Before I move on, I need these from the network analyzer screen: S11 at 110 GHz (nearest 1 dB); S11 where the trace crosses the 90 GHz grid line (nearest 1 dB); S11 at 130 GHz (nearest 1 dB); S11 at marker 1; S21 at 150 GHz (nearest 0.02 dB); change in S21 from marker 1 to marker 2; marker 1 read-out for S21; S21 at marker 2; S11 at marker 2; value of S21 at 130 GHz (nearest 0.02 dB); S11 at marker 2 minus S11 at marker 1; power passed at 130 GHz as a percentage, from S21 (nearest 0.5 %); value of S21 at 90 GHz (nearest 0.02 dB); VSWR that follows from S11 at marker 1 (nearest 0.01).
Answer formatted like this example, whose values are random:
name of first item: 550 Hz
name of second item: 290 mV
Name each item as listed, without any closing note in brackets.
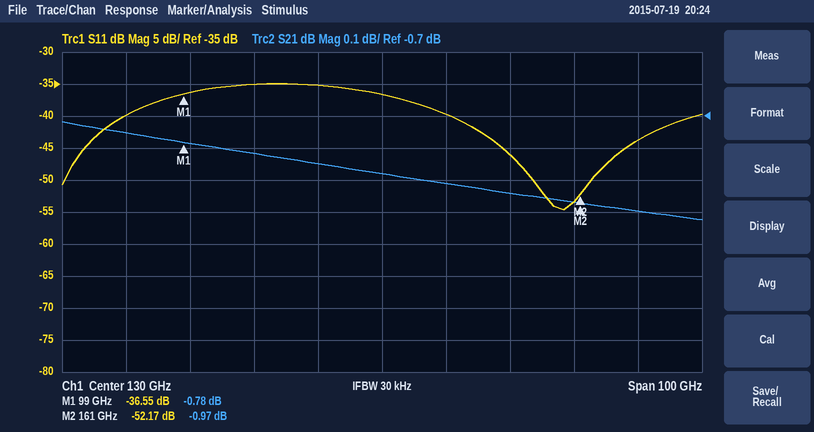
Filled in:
S11 at 110 GHz: -35 dB
S11 where the trace crosses the 90 GHz grid line: -40 dB
S11 at 130 GHz: -37 dB
S11 at marker 1: -36.55 dB
S21 at 150 GHz: -0.94 dB
change in S21 from marker 1 to marker 2: -0.19 dB
marker 1 read-out for S21: -0.78 dB
S21 at marker 2: -0.97 dB
S11 at marker 2: -52.17 dB
value of S21 at 130 GHz: -0.88 dB
S11 at marker 2 minus S11 at marker 1: -15.62 dB
power passed at 130 GHz as a percentage, from S21: 81.5 %
value of S21 at 90 GHz: -0.76 dB
VSWR that follows from S11 at marker 1: 1.03
